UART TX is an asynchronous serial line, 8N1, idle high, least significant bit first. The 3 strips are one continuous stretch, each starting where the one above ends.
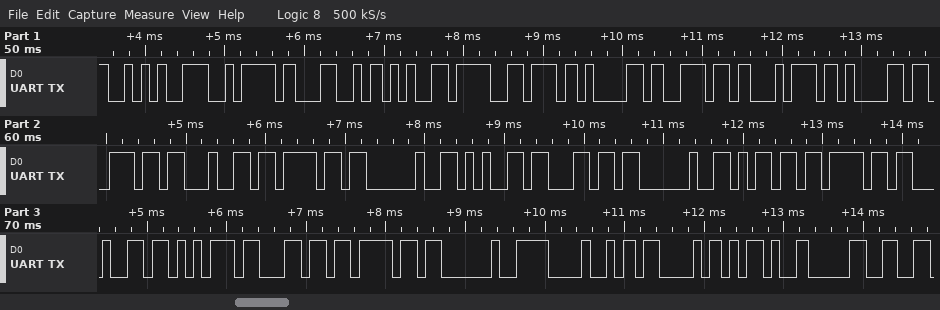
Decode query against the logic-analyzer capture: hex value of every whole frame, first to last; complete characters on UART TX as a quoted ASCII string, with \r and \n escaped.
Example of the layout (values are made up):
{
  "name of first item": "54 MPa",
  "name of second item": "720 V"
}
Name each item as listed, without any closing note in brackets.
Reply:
{
  "hex value of every whole frame, first to last": "2A 7A 4C 65 76 61 6E 74 61 6E 64 6F 20 65 6C 20 6D 6F 64 75 6C 6F 20 48 43 2D 30",
  "complete characters on UART TX as a quoted ASCII string, with \\r and \\n escaped": "\"*zLevantando el modulo HC-0\""
}
